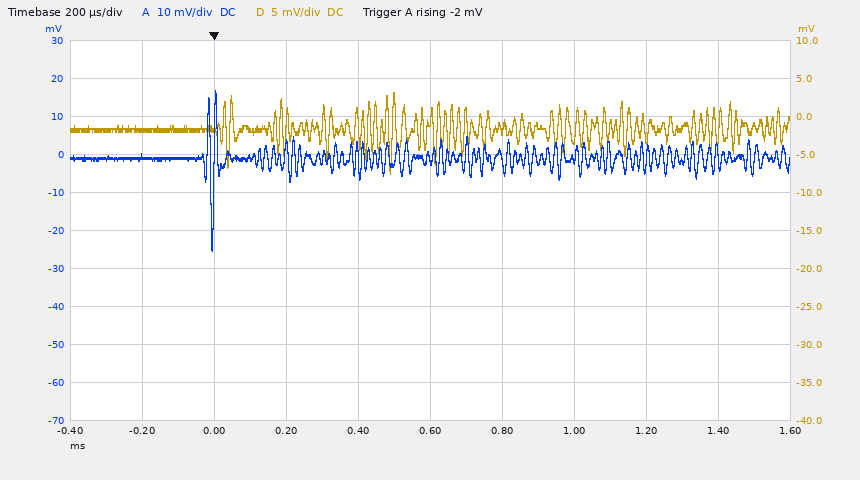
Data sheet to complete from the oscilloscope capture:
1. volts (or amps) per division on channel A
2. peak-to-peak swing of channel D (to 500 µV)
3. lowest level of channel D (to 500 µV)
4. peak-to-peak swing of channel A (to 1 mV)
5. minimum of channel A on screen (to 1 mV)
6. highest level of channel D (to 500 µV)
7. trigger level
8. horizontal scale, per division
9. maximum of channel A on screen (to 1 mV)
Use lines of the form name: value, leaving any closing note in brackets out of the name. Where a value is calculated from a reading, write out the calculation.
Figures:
volts (or amps) per division on channel A: 10 mV
peak-to-peak swing of channel D: 3.0 mV − (-7.5 mV) = 10.5 mV
lowest level of channel D: -7.5 mV
peak-to-peak swing of channel A: 17 mV − (-25 mV) = 42 mV
minimum of channel A on screen: -25 mV
highest level of channel D: 3.0 mV
trigger level: -2 mV
horizontal scale, per division: 200 µs
maximum of channel A on screen: 17 mV
